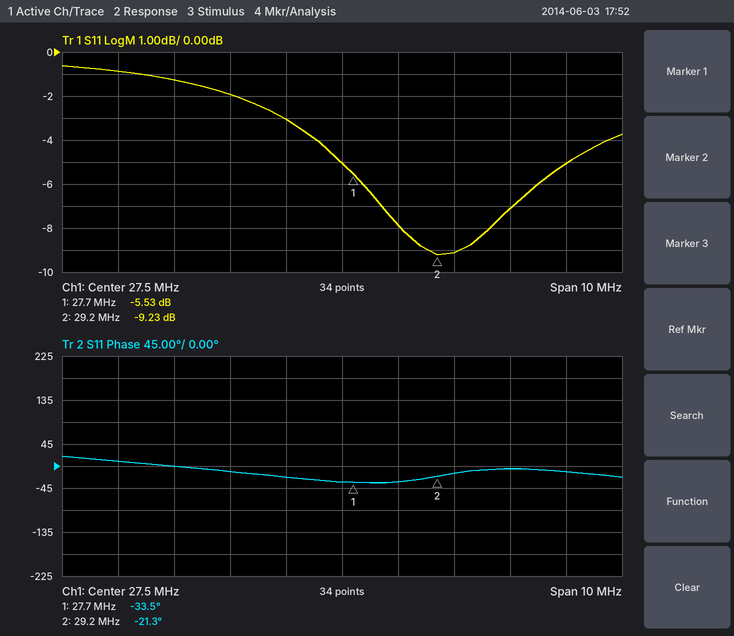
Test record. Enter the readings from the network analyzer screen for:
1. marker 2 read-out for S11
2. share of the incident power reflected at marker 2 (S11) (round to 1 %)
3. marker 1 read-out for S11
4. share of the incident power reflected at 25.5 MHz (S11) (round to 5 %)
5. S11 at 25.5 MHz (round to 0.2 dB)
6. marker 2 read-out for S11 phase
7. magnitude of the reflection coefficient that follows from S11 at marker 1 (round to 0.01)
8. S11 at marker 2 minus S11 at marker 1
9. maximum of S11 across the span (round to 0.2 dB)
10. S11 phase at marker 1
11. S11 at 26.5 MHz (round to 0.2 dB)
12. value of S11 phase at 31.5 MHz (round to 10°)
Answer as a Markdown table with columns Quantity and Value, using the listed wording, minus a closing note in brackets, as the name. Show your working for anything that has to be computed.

| Quantity | Value |
|---|---|
| marker 2 read-out for S11 | -9.23 dB |
| share of the incident power reflected at marker 2 (S11) | 10^(-9.23/10) ≈ 12 % |
| marker 1 read-out for S11 | -5.53 dB |
| share of the incident power reflected at 25.5 MHz (S11) | 10^(-2/10) ≈ 63.1 %, so 65 % to the nearest 5 % |
| S11 at 25.5 MHz | -2.0 dB |
| marker 2 read-out for S11 phase | -21.3° |
| magnitude of the reflection coefficient that follows from S11 at marker 1 | 10^(-5.53/20) ≈ 0.53 |
| S11 at marker 2 minus S11 at marker 1 | -9.23 − (-5.53) = -3.70 dB |
| maximum of S11 across the span | -0.6 dB |
| S11 phase at marker 1 | -33.5° |
| S11 at 26.5 MHz | -3.0 dB |
| value of S11 phase at 31.5 MHz | -10° |
